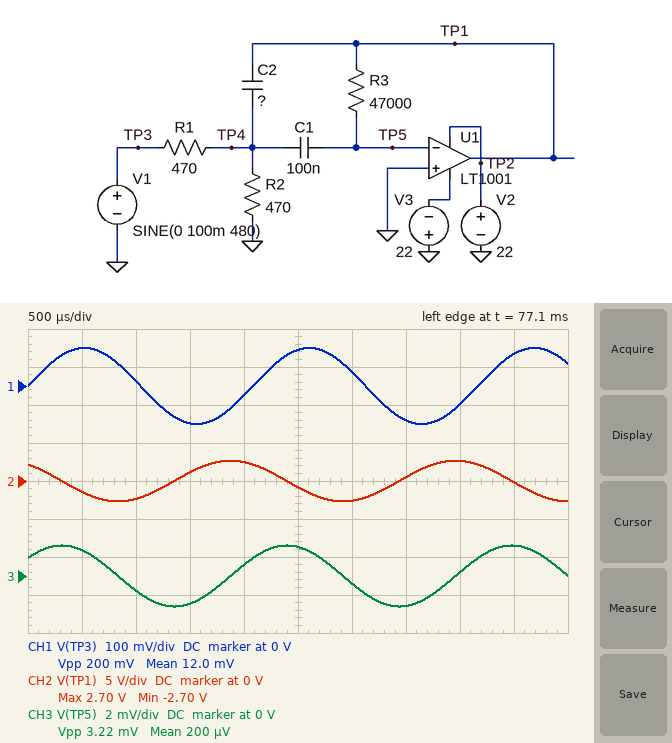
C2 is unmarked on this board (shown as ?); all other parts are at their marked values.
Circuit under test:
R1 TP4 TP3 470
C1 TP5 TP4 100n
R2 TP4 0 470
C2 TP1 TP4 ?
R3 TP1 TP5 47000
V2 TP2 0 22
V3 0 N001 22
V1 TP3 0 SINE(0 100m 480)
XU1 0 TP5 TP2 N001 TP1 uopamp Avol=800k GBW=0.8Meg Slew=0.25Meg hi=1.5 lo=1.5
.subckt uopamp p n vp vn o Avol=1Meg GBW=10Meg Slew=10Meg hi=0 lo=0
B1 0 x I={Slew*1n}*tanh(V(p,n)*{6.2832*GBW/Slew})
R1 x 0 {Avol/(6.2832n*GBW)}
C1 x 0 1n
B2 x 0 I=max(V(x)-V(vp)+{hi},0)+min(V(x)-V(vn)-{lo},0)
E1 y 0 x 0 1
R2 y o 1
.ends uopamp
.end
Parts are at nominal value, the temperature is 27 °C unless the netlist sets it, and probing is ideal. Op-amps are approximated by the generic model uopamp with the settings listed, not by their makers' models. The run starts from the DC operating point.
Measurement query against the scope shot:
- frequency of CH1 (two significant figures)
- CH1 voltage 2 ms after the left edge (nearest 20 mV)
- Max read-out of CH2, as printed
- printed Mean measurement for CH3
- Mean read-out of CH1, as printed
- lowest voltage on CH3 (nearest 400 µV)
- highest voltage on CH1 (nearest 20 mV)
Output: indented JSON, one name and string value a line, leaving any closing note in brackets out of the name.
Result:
{
  "frequency of CH1": "480 Hz",
  "CH1 voltage 2 ms after the left edge": "-20 mV",
  "Max read-out of CH2, as printed": "2.70 V",
  "printed Mean measurement for CH3": "200 µV",
  "Mean read-out of CH1, as printed": "12.0 mV",
  "lowest voltage on CH3": "-1.6 mV",
  "highest voltage on CH1": "100 mV"
}
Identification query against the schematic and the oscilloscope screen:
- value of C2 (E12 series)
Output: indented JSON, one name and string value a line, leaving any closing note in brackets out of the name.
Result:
{
  "value of C2": "120 nF"
}
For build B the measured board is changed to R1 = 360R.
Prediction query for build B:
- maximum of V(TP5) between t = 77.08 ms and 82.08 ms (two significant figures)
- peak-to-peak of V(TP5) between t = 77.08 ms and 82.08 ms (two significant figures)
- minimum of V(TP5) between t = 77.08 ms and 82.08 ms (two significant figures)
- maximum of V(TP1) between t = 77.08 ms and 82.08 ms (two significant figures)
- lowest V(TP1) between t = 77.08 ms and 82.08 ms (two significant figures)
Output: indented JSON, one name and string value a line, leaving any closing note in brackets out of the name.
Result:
{
  "maximum of V(TP5) between t = 77.08 ms and 82.08 ms": "3.3 mV",
  "peak-to-peak of V(TP5) between t = 77.08 ms and 82.08 ms": "6.6 mV",
  "minimum of V(TP5) between t = 77.08 ms and 82.08 ms": "-3.3 mV",
  "maximum of V(TP1) between t = 77.08 ms and 82.08 ms": "5.5 V",
  "lowest V(TP1) between t = 77.08 ms and 82.08 ms": "-5.5 V"
}
